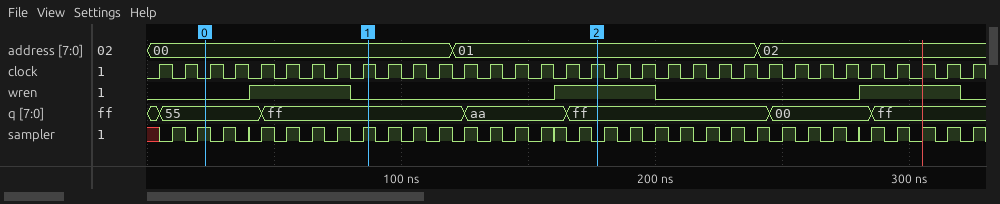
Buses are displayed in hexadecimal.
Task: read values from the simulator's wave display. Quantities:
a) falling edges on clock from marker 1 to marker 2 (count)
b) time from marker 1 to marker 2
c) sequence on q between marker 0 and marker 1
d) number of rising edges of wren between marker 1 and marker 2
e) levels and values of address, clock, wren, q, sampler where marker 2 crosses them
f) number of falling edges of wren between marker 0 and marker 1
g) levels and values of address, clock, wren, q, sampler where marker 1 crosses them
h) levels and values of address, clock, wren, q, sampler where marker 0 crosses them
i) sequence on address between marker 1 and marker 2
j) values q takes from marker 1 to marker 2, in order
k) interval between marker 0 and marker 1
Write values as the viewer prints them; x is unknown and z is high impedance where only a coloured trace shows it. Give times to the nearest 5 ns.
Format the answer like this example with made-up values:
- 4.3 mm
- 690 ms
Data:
- 9
- 90 ns
- 55, ff
- 1
- address=01, clock=1, wren=1, q=ff, sampler=0
- 1
- address=00, clock=1, wren=0, q=ff, sampler=1
- address=00, clock=0, wren=0, q=55, sampler=1
- 00, 01
- ff, aa, ff
- 65 ns
